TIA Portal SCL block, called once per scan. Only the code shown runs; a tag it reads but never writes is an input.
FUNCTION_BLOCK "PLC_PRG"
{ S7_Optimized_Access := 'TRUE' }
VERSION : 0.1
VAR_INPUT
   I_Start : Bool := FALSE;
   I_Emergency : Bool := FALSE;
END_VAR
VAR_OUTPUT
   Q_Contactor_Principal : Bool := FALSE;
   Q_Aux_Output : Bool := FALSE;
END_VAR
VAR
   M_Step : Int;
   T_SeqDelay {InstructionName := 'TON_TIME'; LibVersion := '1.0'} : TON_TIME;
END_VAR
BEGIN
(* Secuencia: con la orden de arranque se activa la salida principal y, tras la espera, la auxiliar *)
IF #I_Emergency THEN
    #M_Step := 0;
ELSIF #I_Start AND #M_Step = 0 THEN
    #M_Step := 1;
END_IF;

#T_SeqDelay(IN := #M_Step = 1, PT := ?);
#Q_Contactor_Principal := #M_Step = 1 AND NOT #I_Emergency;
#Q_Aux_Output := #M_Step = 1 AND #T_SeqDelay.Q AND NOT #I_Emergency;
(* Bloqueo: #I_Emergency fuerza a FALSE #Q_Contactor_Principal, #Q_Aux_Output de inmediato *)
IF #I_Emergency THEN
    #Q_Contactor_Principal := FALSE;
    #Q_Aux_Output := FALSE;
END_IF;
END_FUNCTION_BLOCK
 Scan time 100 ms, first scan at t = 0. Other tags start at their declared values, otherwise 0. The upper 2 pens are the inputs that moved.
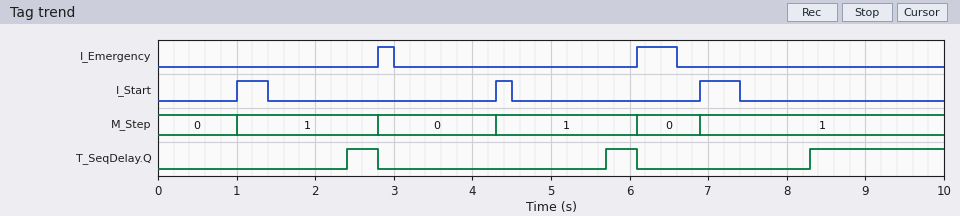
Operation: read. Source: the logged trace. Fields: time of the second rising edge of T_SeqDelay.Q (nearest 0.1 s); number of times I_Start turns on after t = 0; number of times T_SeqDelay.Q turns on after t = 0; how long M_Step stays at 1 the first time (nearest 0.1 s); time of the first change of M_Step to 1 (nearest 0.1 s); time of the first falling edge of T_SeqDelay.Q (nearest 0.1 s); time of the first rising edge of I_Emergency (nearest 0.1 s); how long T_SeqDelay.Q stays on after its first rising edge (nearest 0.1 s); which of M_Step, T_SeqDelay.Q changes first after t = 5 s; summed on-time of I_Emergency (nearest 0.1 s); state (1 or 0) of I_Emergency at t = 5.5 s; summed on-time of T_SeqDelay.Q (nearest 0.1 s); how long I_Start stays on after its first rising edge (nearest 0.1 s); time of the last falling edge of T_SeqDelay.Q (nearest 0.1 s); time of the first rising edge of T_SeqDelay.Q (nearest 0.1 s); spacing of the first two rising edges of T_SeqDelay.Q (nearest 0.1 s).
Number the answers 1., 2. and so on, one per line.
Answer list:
1. 5.7 s
2. 3
3. 3
4. 1.8 s
5. 1.0 s
6. 2.8 s
7. 2.8 s
8. 0.4 s
9. T_SeqDelay.Q
10. 0.7 s
11. 0
12. 2.5 s
13. 0.4 s
14. 6.1 s
15. 2.4 s
16. 3.3 s
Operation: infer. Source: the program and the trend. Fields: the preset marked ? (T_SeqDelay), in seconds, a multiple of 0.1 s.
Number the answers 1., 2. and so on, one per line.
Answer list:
1. 1.4 s
